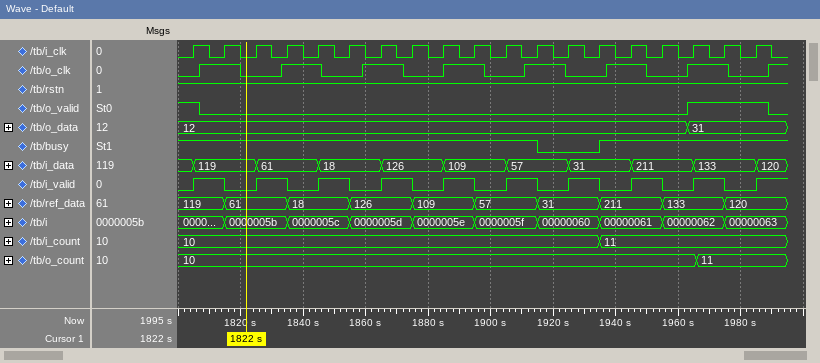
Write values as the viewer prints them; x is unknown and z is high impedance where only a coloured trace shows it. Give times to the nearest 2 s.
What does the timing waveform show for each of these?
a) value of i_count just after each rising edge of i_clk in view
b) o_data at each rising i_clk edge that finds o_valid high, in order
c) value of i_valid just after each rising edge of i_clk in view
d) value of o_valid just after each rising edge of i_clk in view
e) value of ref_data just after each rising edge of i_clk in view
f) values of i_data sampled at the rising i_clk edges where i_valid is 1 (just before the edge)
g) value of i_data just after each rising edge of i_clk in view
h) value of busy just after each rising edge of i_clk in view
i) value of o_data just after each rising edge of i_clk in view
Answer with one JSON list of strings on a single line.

["10, 10, 10, 10, 10, 10, 10, 10, 10, 10, 10, 10, 10, 11, 11, 11, 11, 11, 11", "12, 31, 31, 31", "1 0 1 0 1 0 1 0 1 0 1 0 1 0 1 0 1 0 1", "1 0 0 0 0 0 0 0 0 0 0 0 0 0 0 0 1 1 1", "119, 61, 61, 18, 18, 126, 126, 109, 109, 57, 57, 31, 31, 211, 211, 133, 133, 120, 120", "119, 61, 18, 126, 109, 57, 31, 211, 133", "119, 119, 61, 61, 18, 18, 126, 126, 109, 109, 57, 57, 31, 31, 211, 211, 133, 133, 120", "1 1 1 1 1 1 1 1 1 1 1 0 0 1 1 1 1 1 1", "12, 12, 12, 12, 12, 12, 12, 12, 12, 12, 12, 12, 12, 12, 12, 12, 31, 31, 31"]
